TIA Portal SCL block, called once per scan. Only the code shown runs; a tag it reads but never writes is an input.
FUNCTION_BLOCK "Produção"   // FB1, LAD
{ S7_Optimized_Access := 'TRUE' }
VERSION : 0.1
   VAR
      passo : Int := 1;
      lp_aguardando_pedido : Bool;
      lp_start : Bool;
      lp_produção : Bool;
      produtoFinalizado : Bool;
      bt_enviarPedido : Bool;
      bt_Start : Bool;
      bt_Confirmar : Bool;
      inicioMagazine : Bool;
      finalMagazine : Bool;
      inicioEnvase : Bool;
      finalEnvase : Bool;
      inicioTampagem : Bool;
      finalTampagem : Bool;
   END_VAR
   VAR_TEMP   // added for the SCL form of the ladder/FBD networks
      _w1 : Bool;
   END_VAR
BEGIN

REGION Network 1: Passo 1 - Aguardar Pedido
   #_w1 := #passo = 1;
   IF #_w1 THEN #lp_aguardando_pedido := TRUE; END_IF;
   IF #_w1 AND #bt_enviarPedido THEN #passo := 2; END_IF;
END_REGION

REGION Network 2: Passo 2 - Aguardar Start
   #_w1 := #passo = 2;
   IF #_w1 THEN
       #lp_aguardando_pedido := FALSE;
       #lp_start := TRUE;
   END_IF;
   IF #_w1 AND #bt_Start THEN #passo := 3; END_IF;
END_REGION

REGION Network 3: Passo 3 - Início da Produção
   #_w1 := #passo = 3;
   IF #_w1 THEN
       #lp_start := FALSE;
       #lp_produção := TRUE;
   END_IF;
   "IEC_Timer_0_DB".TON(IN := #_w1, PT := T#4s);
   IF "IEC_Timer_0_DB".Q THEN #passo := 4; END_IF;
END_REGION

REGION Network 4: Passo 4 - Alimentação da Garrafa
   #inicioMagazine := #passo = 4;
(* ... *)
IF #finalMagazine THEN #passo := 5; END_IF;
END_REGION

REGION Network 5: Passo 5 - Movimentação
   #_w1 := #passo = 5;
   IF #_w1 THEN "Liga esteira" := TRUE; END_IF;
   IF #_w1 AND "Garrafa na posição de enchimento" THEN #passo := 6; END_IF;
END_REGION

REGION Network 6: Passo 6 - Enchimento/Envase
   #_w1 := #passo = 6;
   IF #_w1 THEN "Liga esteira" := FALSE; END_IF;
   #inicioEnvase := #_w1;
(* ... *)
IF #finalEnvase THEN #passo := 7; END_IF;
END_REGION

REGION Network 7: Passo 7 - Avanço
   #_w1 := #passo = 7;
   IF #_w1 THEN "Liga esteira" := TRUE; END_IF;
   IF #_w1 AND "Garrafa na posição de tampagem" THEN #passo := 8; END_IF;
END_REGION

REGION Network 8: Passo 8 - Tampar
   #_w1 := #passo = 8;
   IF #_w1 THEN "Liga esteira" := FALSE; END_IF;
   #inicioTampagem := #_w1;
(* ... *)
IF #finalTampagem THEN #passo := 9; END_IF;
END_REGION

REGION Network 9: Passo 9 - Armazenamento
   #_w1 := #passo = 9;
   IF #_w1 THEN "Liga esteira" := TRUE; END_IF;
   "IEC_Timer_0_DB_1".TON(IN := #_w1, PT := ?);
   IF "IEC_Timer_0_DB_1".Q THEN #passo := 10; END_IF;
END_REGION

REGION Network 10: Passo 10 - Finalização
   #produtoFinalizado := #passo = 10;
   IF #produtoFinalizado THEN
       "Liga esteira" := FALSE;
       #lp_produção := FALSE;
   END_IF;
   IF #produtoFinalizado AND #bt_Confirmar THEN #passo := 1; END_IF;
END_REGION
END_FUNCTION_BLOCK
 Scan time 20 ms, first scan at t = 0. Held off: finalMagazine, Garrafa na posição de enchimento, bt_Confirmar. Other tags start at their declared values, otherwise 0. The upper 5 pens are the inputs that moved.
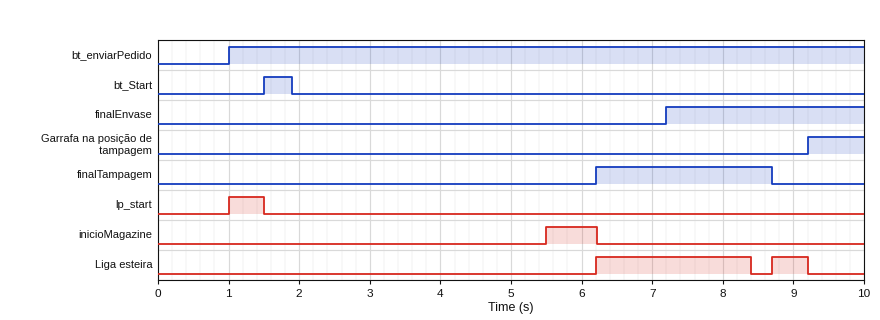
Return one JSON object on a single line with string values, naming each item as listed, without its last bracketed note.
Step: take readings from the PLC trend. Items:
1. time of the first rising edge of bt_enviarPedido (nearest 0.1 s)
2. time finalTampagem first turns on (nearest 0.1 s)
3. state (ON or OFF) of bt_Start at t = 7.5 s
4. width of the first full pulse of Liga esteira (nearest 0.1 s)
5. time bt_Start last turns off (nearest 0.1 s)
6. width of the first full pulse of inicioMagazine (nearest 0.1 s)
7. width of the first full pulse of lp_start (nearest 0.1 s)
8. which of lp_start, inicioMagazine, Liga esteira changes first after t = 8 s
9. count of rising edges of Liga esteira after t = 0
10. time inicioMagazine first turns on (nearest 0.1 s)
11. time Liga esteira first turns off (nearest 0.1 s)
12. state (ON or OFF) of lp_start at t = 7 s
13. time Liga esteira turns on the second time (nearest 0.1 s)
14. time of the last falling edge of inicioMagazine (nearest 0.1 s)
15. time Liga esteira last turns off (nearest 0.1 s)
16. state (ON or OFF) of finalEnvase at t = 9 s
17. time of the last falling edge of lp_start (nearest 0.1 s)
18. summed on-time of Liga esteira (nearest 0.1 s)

{"time of the first rising edge of bt_enviarPedido": "1.0 s", "time finalTampagem first turns on": "6.2 s", "state (ON or OFF) of bt_Start at t = 7.5 s": "OFF", "width of the first full pulse of Liga esteira": "2.2 s", "time bt_Start last turns off": "1.9 s", "width of the first full pulse of inicioMagazine": "0.7 s", "width of the first full pulse of lp_start": "0.5 s", "which of lp_start, inicioMagazine, Liga esteira changes first after t = 8 s": "Liga esteira", "count of rising edges of Liga esteira after t = 0": "2", "time inicioMagazine first turns on": "5.5 s", "time Liga esteira first turns off": "8.4 s", "state (ON or OFF) of lp_start at t = 7 s": "OFF", "time Liga esteira turns on the second time": "8.7 s", "time of the last falling edge of inicioMagazine": "6.2 s", "time Liga esteira last turns off": "9.2 s", "state (ON or OFF) of finalEnvase at t = 9 s": "ON", "time of the last falling edge of lp_start": "1.5 s", "summed on-time of Liga esteira": "2.7 s"}
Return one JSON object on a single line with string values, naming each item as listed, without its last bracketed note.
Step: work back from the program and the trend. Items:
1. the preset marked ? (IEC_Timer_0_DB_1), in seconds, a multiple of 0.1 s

{"the preset marked ? (IEC_Timer_0_DB_1), in seconds, a multiple of 0.1 s": "2.2 s"}
